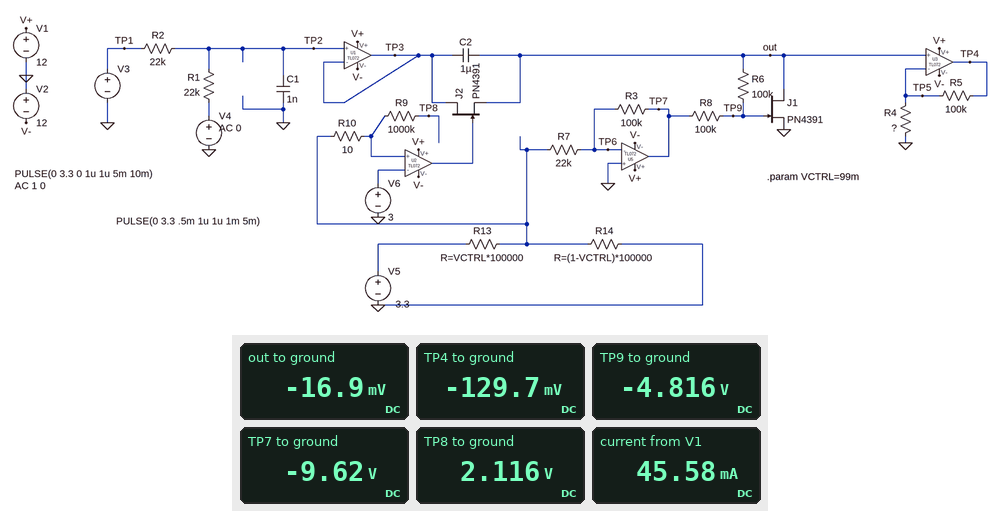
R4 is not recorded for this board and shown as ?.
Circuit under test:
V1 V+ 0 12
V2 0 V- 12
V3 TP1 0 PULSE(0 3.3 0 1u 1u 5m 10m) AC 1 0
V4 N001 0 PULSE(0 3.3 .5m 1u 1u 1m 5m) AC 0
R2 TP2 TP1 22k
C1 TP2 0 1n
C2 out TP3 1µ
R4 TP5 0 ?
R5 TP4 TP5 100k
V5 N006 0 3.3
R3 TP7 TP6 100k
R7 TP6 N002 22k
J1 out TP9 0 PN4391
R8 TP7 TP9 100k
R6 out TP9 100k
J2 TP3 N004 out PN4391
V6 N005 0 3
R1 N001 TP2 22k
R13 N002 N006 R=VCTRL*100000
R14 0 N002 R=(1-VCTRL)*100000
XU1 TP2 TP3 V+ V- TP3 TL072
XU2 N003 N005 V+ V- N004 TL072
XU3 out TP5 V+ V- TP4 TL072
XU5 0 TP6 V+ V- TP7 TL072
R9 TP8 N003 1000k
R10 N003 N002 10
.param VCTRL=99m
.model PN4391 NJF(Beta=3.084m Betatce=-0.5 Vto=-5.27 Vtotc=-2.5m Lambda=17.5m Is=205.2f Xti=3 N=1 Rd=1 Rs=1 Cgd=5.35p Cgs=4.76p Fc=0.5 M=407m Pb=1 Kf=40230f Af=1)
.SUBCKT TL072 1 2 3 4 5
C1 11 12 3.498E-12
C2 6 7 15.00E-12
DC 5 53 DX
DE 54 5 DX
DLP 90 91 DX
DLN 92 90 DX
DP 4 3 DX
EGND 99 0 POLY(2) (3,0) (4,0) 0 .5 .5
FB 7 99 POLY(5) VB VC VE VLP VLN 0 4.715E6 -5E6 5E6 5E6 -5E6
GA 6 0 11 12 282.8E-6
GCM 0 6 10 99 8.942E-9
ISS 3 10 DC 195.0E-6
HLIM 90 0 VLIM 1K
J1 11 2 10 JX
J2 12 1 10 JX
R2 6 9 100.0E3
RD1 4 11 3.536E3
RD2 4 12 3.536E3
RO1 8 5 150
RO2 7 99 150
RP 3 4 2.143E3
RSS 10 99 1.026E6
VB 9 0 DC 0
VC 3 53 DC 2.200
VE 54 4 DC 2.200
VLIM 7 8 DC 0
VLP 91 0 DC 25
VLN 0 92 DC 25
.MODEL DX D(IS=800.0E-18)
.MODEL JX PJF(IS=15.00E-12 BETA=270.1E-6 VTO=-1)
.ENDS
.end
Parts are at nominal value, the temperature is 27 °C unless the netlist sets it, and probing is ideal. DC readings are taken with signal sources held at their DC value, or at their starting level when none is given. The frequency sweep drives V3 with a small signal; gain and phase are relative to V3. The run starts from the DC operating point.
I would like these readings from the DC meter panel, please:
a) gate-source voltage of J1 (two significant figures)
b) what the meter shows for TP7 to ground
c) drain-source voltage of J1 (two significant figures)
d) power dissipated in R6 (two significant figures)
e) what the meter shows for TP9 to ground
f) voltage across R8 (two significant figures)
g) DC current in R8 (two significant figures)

-4.8 V
-9.62 V
-17 mV
230 µW
-4.816 V
4.8 V
48 µA
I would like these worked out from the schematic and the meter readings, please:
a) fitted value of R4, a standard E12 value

15 kΩ
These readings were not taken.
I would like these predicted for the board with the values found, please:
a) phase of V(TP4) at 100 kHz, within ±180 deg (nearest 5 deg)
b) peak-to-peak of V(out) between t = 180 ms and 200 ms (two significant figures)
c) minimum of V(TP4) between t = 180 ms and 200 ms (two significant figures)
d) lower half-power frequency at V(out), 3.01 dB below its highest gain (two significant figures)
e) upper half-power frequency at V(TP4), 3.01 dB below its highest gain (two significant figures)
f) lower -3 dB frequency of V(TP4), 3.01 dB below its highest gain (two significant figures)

-95 deg
3.3 V
-10 V
430 Hz
15 kHz
430 Hz
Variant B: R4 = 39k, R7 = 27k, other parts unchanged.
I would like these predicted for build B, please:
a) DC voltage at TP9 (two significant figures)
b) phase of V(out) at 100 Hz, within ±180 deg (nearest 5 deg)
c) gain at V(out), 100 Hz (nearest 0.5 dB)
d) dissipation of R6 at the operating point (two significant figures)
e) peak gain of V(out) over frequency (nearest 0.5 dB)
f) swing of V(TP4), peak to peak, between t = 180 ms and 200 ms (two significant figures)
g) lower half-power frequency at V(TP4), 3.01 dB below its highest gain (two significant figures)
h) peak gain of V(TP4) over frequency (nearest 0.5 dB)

-4.1 V
85 deg
-27.0 dB
170 µW
-6.5 dB
9.7 V
960 Hz
4.5 dB
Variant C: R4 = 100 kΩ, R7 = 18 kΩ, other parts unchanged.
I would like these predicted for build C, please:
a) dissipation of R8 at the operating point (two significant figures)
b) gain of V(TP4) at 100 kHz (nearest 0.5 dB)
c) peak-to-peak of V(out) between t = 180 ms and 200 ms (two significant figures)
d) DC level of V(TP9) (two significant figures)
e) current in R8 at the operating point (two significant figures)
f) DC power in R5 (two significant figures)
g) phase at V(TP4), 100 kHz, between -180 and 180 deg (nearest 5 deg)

260 µW
-17.0 dB
4.1 V
-5.3 V
51 µA
240 nW
-85 deg
